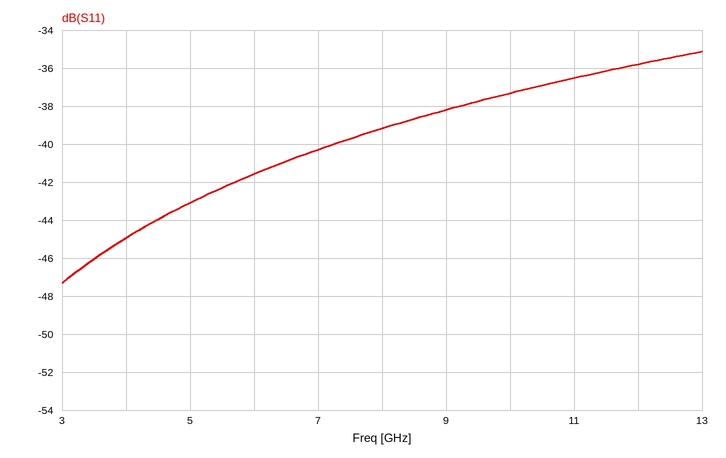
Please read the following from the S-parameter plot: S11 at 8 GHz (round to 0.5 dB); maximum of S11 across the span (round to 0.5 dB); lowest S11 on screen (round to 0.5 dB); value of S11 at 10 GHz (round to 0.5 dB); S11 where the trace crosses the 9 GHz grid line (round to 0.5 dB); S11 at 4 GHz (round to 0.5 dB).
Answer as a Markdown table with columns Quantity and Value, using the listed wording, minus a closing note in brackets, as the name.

| Quantity | Value |
|---|---|
| S11 at 8 GHz | -39.0 dB |
| maximum of S11 across the span | -35.0 dB |
| lowest S11 on screen | -47.5 dB |
| value of S11 at 10 GHz | -37.5 dB |
| S11 where the trace crosses the 9 GHz grid line | -38.0 dB |
| S11 at 4 GHz | -45.0 dB |
